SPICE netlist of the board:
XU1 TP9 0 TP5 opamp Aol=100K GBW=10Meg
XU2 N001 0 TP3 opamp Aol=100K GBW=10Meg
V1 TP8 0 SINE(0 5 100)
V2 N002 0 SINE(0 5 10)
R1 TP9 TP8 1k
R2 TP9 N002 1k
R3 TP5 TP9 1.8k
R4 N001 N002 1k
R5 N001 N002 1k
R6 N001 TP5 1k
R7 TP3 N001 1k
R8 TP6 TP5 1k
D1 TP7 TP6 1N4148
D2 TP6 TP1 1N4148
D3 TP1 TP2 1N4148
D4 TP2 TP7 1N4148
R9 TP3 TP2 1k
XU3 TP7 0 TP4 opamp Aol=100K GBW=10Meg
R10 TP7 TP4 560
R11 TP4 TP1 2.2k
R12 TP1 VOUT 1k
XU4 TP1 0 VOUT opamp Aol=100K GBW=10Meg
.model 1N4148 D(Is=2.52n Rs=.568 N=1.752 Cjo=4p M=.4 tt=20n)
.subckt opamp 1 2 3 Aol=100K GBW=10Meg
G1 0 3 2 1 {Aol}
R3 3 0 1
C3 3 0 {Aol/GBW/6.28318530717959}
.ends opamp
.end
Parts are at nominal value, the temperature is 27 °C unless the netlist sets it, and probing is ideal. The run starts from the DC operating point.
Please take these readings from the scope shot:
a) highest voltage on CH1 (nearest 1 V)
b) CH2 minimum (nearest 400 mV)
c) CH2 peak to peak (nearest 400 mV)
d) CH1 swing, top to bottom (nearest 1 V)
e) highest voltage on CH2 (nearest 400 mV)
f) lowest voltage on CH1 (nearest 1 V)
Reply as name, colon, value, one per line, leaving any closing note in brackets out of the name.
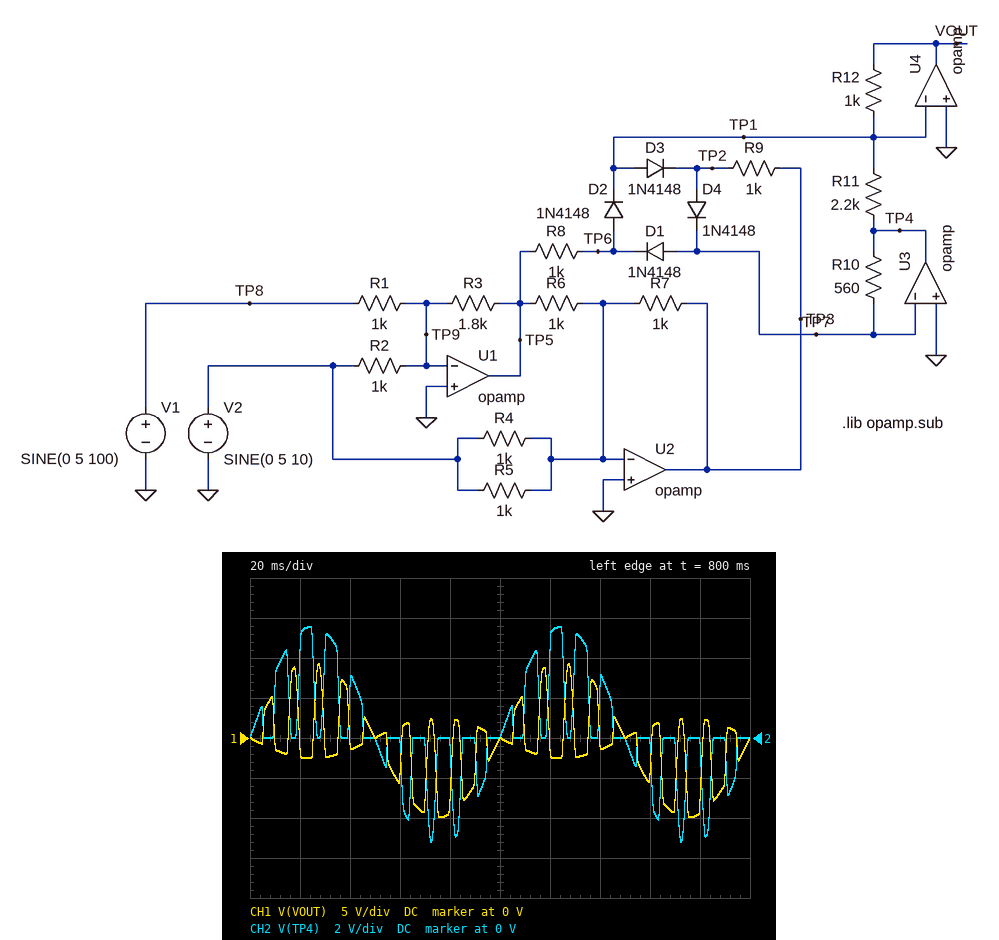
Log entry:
highest voltage on CH1: 9 V
CH2 minimum: -5.2 V
CH2 peak to peak: 10.8 V
CH1 swing, top to bottom: 19 V
highest voltage on CH2: 5.6 V
lowest voltage on CH1: -10 V
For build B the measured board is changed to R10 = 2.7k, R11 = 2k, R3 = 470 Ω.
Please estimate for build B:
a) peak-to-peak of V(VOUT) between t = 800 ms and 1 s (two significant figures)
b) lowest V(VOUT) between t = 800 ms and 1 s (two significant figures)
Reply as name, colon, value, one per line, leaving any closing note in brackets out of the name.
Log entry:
peak-to-peak of V(VOUT) between t = 800 ms and 1 s: 16 V
lowest V(VOUT) between t = 800 ms and 1 s: -3.2 V
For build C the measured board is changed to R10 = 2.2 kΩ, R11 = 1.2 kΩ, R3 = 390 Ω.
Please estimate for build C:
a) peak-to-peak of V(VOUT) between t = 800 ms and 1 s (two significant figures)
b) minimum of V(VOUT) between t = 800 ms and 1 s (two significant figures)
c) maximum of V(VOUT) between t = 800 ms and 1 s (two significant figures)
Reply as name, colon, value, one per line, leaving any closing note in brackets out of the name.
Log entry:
peak-to-peak of V(VOUT) between t = 800 ms and 1 s: 20 V
minimum of V(VOUT) between t = 800 ms and 1 s: -3.0 V
maximum of V(VOUT) between t = 800 ms and 1 s: 17 V
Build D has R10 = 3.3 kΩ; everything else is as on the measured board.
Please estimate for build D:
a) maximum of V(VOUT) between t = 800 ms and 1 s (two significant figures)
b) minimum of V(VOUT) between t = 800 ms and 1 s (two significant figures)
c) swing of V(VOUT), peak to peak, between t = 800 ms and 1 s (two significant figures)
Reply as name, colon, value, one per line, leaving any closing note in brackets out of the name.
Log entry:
maximum of V(VOUT) between t = 800 ms and 1 s: 14 V
minimum of V(VOUT) between t = 800 ms and 1 s: -15 V
swing of V(VOUT), peak to peak, between t = 800 ms and 1 s: 29 V
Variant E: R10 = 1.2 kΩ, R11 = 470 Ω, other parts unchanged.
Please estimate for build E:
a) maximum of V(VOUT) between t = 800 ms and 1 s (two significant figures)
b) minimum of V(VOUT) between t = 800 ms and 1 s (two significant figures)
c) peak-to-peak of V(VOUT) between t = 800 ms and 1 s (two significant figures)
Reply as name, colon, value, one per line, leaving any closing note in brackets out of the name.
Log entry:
maximum of V(VOUT) between t = 800 ms and 1 s: 24 V
minimum of V(VOUT) between t = 800 ms and 1 s: -25 V
peak-to-peak of V(VOUT) between t = 800 ms and 1 s: 49 V
